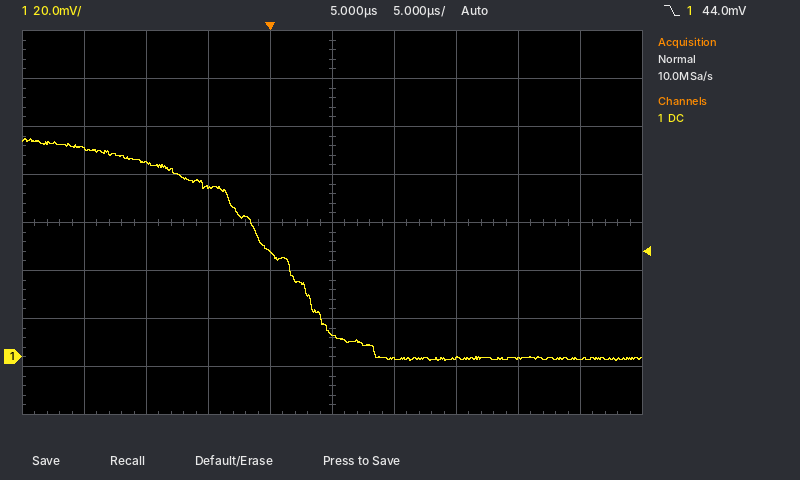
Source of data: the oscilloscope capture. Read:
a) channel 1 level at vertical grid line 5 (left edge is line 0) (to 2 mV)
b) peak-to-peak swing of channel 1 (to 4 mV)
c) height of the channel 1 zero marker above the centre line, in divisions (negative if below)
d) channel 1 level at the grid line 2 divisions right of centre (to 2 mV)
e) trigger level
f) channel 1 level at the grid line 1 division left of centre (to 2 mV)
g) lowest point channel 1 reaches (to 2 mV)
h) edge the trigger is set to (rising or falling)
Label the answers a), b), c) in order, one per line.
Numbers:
a) 10 mV
b) 92 mV
c) -2.8 div
d) 0 mV
e) 44.0 mV
f) 44 mV
g) -2 mV
h) falling
